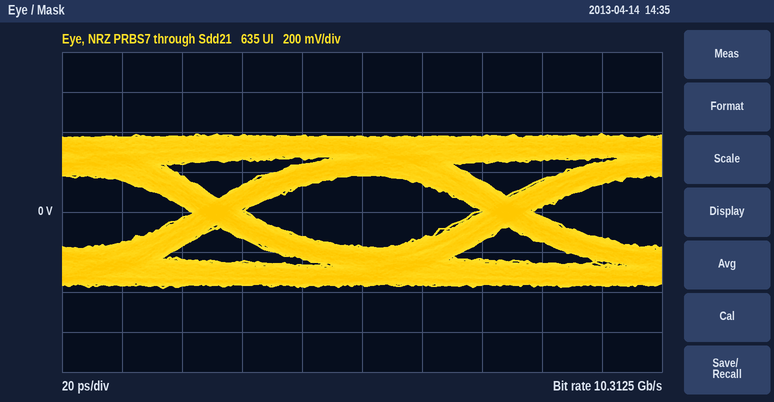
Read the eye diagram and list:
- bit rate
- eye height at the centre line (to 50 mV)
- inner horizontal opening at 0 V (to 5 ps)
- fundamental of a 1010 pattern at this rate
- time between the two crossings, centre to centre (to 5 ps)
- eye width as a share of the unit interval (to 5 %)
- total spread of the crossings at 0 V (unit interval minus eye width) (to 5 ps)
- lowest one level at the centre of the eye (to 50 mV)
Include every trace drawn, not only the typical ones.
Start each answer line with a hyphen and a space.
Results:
- 10.3125 Gb/s
- 350 mV
- 75 ps
- 5.15625 GHz
- 95 ps
- 80 %
- 20 ps
- 200 mV
